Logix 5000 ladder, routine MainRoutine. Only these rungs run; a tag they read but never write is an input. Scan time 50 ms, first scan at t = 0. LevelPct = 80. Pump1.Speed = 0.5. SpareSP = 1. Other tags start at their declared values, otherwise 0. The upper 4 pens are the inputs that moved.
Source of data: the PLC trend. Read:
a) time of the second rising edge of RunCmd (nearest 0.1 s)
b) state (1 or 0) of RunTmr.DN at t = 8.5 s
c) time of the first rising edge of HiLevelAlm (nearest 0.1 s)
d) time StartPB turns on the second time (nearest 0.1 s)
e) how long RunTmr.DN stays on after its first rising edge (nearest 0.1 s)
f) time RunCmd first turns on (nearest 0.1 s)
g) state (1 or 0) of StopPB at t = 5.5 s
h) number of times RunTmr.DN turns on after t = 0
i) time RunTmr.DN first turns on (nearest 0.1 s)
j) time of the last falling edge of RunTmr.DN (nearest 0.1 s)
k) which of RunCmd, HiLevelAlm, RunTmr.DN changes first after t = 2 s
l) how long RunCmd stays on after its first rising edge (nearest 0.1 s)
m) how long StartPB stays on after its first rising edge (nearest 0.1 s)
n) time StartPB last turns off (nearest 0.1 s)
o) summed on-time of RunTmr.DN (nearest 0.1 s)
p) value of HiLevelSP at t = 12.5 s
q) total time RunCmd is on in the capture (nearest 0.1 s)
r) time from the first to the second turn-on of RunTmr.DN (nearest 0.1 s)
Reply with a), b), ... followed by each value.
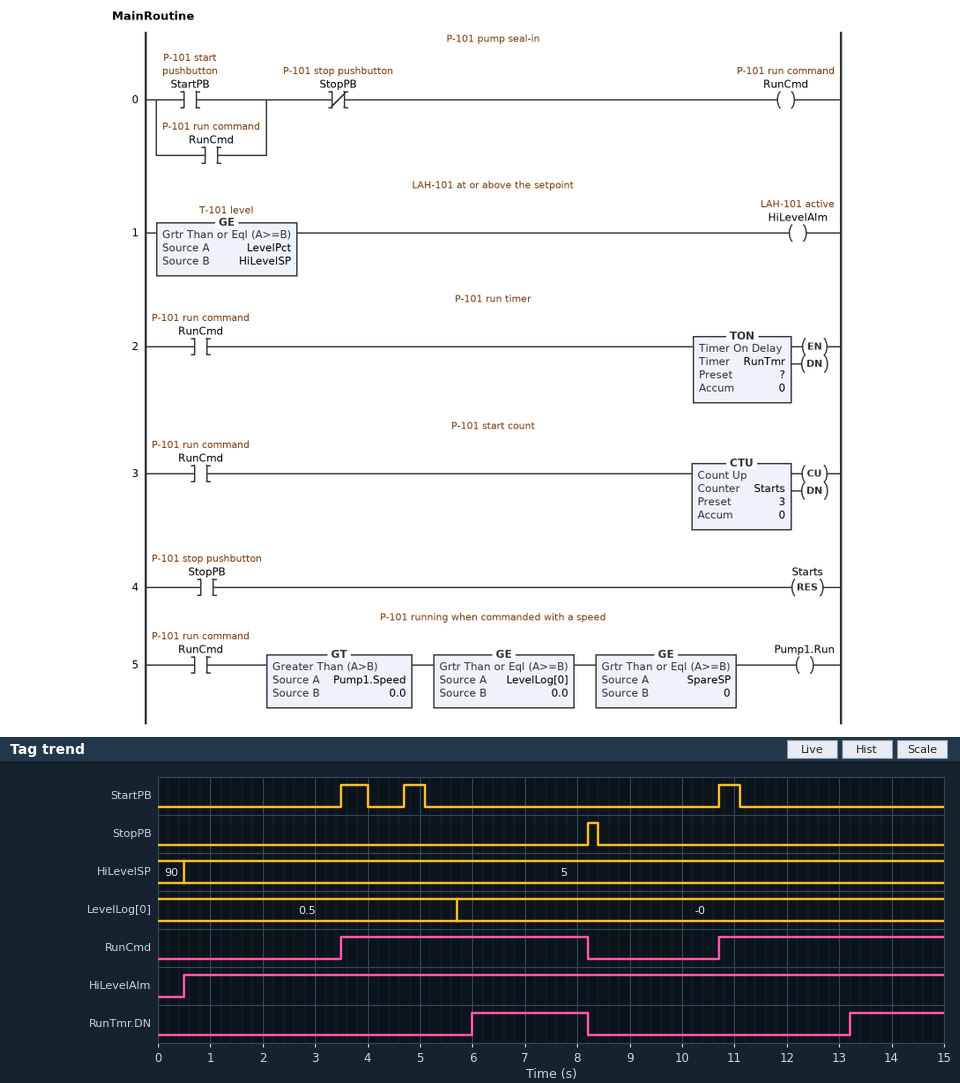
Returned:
a) 10.7 s
b) 0
c) 0.5 s
d) 4.7 s
e) 2.2 s
f) 3.5 s
g) 0
h) 2
i) 6.0 s
j) 8.2 s
k) RunCmd
l) 4.7 s
m) 0.5 s
n) 11.1 s
o) 4.0 s
p) 5
q) 9.0 s
r) 7.2 s
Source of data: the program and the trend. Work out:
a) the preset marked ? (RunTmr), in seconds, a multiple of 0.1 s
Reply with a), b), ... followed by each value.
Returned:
a) 2.5 s
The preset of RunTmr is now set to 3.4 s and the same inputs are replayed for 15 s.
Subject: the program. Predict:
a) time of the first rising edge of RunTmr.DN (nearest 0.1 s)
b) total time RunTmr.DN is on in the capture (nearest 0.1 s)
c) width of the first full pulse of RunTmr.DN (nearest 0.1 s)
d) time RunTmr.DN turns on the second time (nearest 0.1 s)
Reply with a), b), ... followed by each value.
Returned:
a) 6.9 s
b) 2.2 s
c) 1.3 s
d) 14.1 s
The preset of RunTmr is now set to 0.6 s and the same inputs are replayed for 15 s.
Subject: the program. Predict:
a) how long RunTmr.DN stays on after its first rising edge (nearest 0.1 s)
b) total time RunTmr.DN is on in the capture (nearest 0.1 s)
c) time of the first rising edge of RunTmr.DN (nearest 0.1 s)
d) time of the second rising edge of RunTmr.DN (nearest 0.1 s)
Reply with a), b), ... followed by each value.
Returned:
a) 4.1 s
b) 7.8 s
c) 4.1 s
d) 11.3 s
